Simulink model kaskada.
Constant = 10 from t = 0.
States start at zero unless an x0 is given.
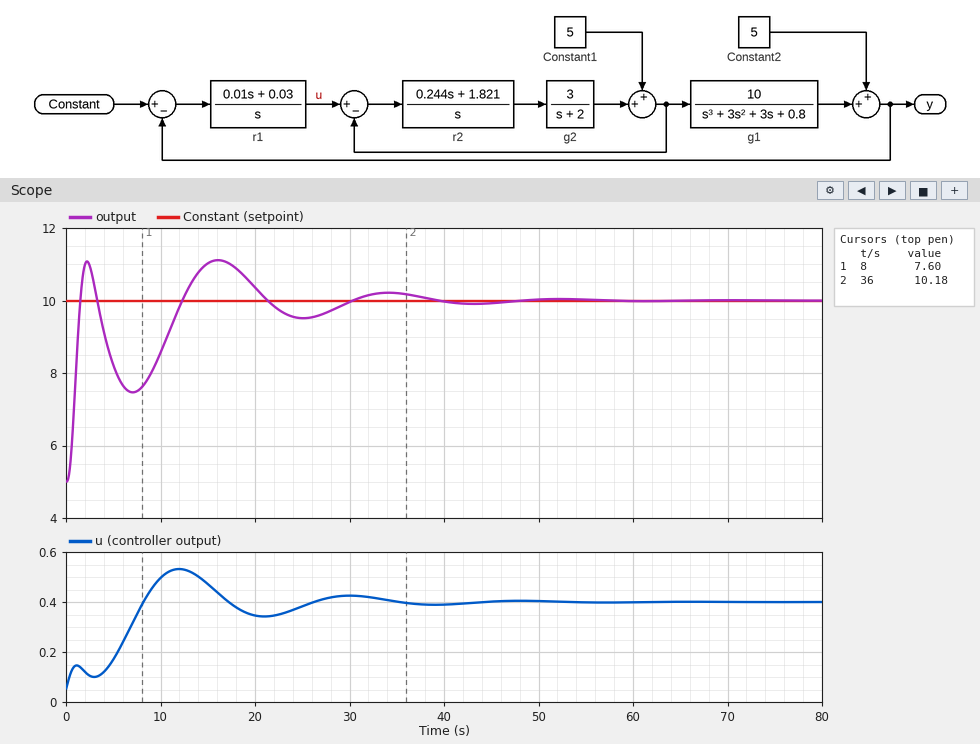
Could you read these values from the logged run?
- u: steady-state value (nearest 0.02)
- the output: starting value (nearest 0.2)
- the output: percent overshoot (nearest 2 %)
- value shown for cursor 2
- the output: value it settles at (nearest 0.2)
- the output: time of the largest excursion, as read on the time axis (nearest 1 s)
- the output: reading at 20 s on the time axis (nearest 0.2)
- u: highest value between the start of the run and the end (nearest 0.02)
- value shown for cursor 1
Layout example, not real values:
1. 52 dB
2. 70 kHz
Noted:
1. 0.40
2. 5.0
3. 22 %
4. 10.18
5. 10.0
6. 16 s
7. 10.4
8. 0.54
9. 7.60
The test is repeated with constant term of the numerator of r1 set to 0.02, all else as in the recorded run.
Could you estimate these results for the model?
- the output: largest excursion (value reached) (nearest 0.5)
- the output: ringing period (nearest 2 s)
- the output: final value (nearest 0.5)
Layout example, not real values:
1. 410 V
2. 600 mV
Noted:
1. 11.0
2. 16 s
3. 10.0
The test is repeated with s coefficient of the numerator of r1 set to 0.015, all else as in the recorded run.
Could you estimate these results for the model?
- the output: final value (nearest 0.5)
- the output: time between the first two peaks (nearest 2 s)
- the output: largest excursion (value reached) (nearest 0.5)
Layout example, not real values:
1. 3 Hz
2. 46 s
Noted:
1. 10.0
2. 14 s
3. 11.0
